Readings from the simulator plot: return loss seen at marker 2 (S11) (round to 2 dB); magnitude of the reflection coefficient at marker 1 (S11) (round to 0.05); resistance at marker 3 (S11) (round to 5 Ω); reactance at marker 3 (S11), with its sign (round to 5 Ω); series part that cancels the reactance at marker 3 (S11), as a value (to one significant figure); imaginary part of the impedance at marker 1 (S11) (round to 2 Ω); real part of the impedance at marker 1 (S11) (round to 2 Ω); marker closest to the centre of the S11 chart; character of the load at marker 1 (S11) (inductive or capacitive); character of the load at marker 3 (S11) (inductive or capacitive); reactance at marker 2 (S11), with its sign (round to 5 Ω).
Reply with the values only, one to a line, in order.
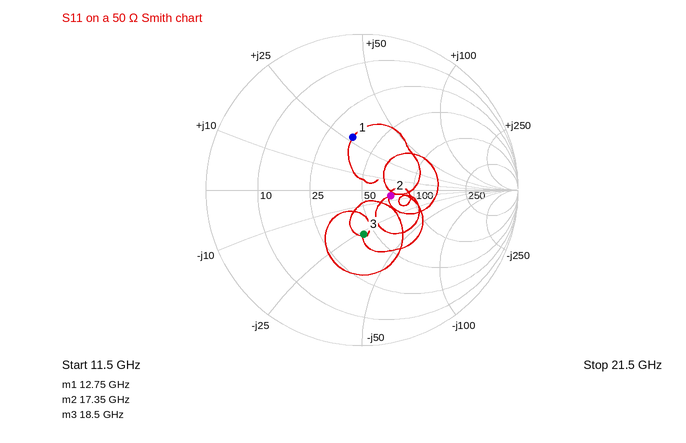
14 dB
0.35
45 Ω
-25 Ω
200 pH
+28 Ω
36 Ω
marker 2
inductive
capacitive
-5 Ω
